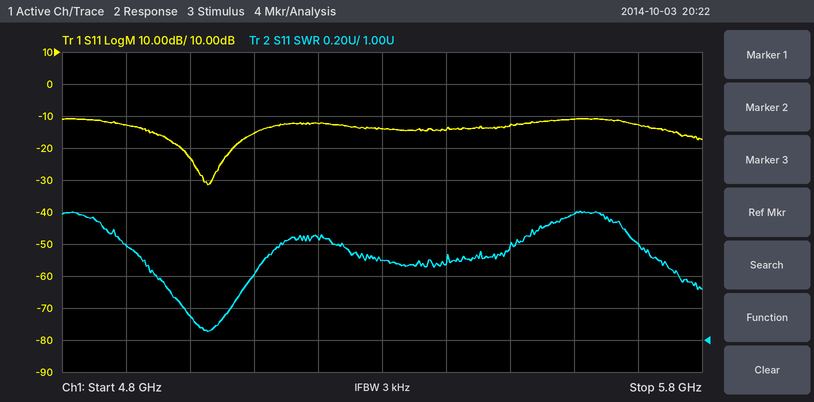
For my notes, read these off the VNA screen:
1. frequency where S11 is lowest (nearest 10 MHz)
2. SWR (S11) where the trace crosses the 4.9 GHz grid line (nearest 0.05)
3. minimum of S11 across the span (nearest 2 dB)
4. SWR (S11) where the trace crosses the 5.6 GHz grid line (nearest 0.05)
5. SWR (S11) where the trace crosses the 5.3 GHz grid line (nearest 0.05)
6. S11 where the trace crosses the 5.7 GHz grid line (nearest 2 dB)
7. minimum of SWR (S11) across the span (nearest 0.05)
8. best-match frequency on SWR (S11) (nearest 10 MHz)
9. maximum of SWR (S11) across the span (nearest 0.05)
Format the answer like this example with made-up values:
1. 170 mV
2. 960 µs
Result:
1. 5.03 GHz
2. 1.60
3. -32 dB
4. 1.80
5. 1.50
6. -12 dB
7. 1.05
8. 5.03 GHz
9. 1.80
